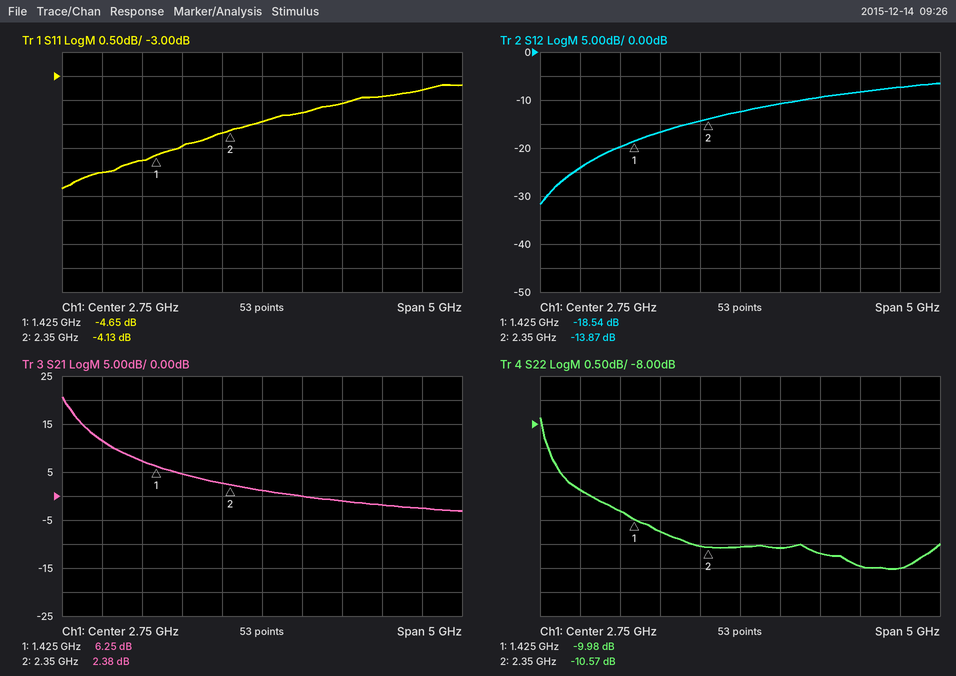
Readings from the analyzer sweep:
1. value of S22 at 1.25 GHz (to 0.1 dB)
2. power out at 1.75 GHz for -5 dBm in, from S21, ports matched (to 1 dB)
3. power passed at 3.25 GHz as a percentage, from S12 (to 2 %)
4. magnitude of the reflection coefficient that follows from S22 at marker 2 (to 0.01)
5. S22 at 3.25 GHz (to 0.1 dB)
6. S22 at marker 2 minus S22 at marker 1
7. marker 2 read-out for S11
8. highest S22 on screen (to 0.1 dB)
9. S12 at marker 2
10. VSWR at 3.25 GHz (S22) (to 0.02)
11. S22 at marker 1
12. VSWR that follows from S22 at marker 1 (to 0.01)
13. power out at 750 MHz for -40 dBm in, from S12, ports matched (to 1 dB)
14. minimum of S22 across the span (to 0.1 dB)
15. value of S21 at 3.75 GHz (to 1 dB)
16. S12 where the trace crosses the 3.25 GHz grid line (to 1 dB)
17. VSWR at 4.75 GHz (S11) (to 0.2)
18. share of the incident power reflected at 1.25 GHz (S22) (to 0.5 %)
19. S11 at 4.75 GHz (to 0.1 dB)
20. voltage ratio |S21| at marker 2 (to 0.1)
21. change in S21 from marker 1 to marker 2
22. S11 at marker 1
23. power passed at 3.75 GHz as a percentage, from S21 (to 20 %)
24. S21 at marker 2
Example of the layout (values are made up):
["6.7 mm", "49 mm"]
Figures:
["-9.8 dB", "0 dBm", "8 %", "0.30", "-10.6 dB", "-0.59 dB", "-4.13 dB", "-7.9 dB", "-13.87 dB", "1.84", "-9.98 dB", "1.93", "-64 dBm", "-11.0 dB", "-1 dB", "-11 dB", "5.4", "10.5 %", "-3.3 dB", "1.3", "-3.87 dB", "-4.65 dB", "80 %", "2.38 dB"]
